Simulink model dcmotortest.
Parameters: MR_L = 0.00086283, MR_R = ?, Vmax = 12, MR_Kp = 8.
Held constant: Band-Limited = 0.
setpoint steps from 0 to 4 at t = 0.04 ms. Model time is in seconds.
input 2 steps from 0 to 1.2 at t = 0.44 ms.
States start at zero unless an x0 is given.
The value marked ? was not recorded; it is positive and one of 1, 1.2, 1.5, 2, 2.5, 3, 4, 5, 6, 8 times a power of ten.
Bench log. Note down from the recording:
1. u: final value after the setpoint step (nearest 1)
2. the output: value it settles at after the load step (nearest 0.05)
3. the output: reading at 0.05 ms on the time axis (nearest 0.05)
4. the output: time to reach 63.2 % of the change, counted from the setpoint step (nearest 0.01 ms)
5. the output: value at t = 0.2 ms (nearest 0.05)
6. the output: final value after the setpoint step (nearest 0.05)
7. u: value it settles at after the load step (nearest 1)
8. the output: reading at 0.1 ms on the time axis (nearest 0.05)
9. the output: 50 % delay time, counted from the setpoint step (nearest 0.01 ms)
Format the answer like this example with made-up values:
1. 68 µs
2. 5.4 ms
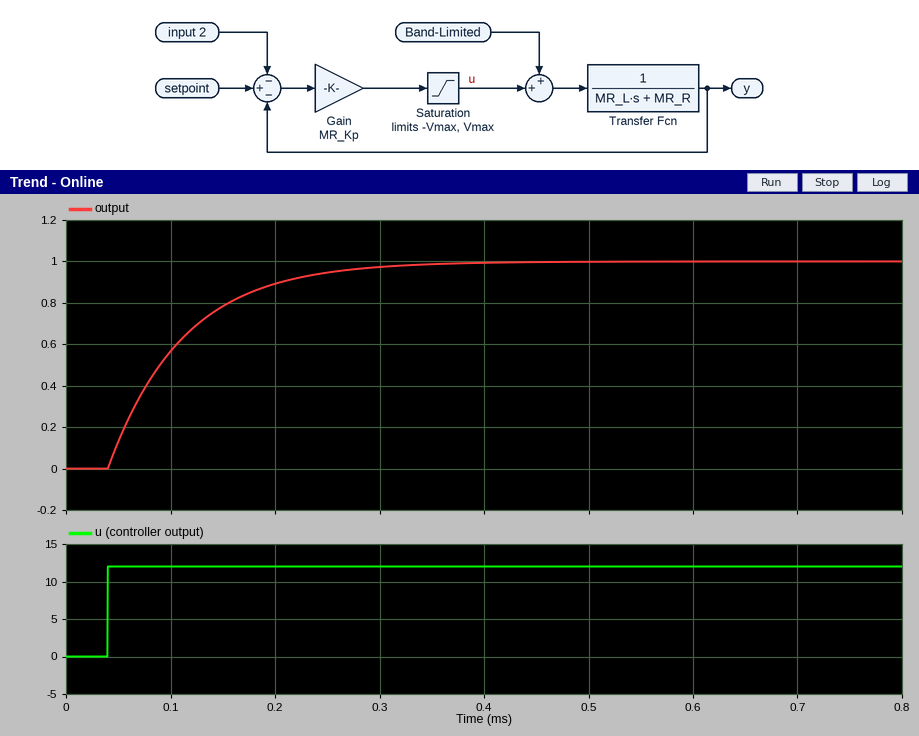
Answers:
1. 12
2. 1.00
3. 0.15
4. 0.07 ms
5. 0.90
6. 1.00
7. 12
8. 0.55
9. 0.05 ms
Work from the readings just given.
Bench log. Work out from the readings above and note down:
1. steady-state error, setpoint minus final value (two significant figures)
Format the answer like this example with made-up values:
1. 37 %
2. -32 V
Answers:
1. 3.0
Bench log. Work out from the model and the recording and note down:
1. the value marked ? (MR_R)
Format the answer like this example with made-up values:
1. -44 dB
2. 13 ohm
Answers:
1. 12
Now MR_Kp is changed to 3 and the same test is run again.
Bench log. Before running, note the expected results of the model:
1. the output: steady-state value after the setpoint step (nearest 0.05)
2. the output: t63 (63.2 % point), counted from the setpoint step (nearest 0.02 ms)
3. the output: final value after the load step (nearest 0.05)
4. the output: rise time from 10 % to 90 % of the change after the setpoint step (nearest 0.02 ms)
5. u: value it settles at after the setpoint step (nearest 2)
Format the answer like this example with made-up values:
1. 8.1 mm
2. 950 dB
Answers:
1. 0.80
2. 0.06 ms
3. 0.55
4. 0.12 ms
5. 10
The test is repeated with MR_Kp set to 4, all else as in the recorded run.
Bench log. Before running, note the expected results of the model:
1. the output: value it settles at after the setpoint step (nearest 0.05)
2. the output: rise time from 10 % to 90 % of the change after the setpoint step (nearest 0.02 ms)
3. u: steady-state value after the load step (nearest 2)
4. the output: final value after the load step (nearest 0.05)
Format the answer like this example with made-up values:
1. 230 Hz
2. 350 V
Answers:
1. 1.00
2. 0.16 ms
3. 8
4. 0.70
